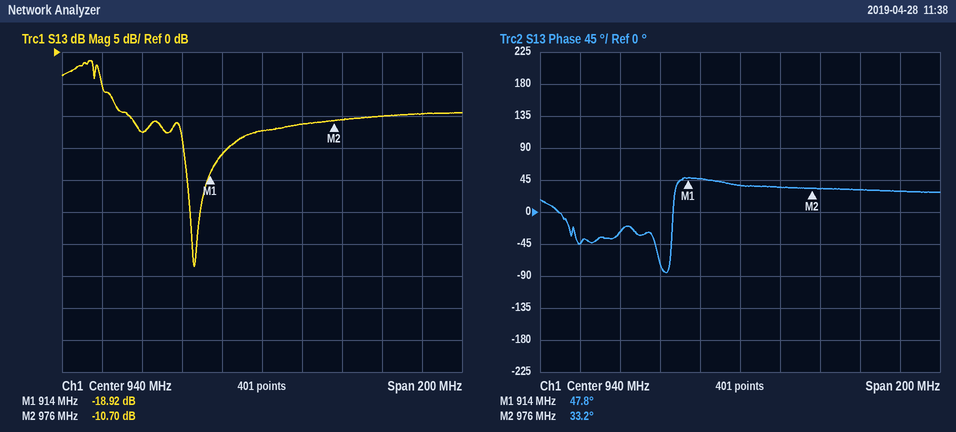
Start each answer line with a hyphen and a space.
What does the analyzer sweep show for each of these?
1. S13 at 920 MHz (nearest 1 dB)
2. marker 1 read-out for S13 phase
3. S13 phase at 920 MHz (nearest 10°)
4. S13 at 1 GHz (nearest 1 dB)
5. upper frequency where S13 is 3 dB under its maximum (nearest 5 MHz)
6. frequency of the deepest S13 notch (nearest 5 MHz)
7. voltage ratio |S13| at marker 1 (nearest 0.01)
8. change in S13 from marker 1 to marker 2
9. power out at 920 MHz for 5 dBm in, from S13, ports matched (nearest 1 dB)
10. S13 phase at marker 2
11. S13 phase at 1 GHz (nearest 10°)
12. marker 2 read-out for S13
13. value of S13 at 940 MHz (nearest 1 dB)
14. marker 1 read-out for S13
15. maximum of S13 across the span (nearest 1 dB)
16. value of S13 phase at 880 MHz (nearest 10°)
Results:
- -16 dB
- 47.8°
- 50°
- -10 dB
- 860 MHz
- 905 MHz
- 0.11
- 8.22 dB
- -11 dBm
- 33.2°
- 30°
- -10.70 dB
- -12 dB
- -18.92 dB
- -1 dB
- -30°
